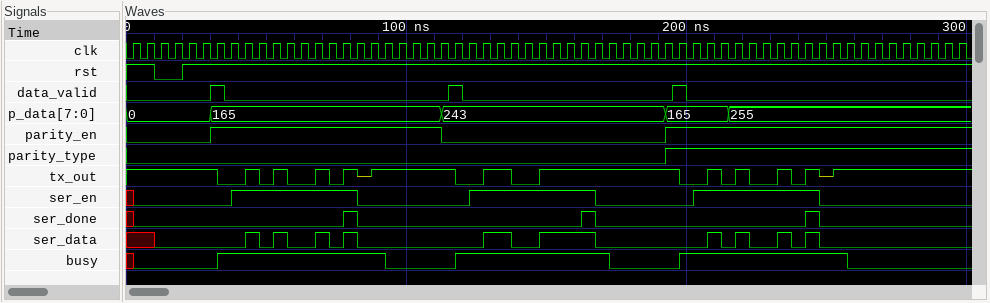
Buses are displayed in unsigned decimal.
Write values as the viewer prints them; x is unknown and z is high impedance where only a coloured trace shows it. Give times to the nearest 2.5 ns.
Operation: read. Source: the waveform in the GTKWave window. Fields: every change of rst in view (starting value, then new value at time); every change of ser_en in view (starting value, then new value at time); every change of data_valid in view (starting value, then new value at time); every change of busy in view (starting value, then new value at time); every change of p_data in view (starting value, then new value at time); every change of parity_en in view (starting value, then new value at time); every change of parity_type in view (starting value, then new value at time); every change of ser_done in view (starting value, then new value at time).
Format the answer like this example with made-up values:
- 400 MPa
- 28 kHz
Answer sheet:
- 1, 0 at 10 ns, 1 at 20 ns
- x, 0 at 2.5 ns, 1 at 37.5 ns, 0 at 82.5 ns, 1 at 122.5 ns, 0 at 167.5 ns, 1 at 202.5 ns, 0 at 247.5 ns
- 0, 1 at 30 ns, 0 at 35 ns, 1 at 115 ns, 0 at 120 ns, 1 at 195 ns, 0 at 200 ns
- x, 0 at 2.5 ns, 1 at 32.5 ns, 0 at 92.5 ns, 1 at 117.5 ns, 0 at 172.5 ns, 1 at 197.5 ns, 0 at 257.5 ns
- 0, 165 at 30 ns, 243 at 112.5 ns, 165 at 192.5 ns, 255 at 215 ns
- 0, 1 at 30 ns, 0 at 112.5 ns, 1 at 192.5 ns
- 0, 1 at 192.5 ns
- x, 0 at 2.5 ns, 1 at 77.5 ns, 0 at 82.5 ns, 1 at 162.5 ns, 0 at 167.5 ns, 1 at 242.5 ns, 0 at 247.5 ns
